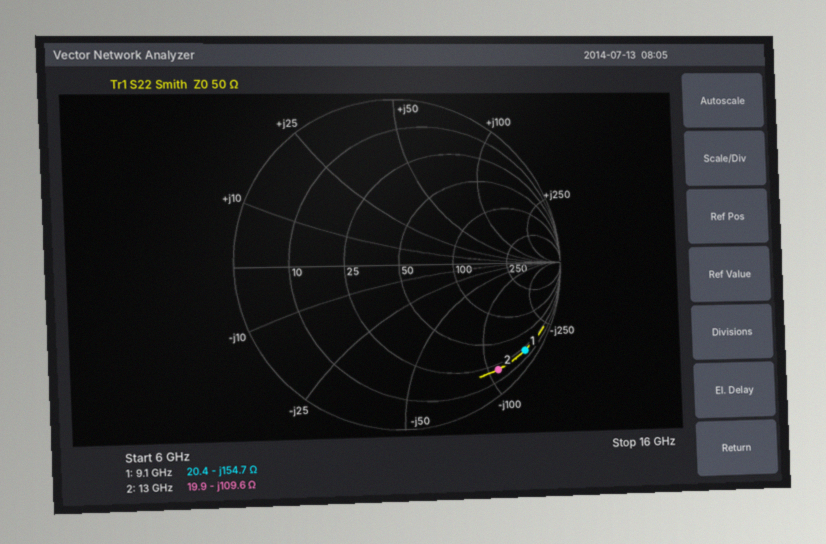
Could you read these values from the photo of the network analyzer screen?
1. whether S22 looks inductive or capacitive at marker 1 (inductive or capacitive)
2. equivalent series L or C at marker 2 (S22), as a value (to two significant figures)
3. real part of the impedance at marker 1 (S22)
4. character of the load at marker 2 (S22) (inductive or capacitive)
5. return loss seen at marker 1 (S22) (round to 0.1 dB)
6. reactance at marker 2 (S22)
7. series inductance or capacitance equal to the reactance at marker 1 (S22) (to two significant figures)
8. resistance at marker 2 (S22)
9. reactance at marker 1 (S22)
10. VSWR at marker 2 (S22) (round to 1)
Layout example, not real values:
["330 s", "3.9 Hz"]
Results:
["capacitive", "110 fF", "20.4 Ω", "capacitive", "0.7 dB", "-109.6 Ω", "110 fF", "19.9 Ω", "-154.7 Ω", "15"]
